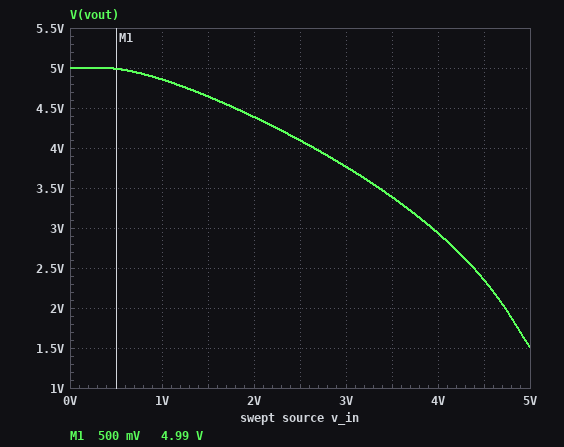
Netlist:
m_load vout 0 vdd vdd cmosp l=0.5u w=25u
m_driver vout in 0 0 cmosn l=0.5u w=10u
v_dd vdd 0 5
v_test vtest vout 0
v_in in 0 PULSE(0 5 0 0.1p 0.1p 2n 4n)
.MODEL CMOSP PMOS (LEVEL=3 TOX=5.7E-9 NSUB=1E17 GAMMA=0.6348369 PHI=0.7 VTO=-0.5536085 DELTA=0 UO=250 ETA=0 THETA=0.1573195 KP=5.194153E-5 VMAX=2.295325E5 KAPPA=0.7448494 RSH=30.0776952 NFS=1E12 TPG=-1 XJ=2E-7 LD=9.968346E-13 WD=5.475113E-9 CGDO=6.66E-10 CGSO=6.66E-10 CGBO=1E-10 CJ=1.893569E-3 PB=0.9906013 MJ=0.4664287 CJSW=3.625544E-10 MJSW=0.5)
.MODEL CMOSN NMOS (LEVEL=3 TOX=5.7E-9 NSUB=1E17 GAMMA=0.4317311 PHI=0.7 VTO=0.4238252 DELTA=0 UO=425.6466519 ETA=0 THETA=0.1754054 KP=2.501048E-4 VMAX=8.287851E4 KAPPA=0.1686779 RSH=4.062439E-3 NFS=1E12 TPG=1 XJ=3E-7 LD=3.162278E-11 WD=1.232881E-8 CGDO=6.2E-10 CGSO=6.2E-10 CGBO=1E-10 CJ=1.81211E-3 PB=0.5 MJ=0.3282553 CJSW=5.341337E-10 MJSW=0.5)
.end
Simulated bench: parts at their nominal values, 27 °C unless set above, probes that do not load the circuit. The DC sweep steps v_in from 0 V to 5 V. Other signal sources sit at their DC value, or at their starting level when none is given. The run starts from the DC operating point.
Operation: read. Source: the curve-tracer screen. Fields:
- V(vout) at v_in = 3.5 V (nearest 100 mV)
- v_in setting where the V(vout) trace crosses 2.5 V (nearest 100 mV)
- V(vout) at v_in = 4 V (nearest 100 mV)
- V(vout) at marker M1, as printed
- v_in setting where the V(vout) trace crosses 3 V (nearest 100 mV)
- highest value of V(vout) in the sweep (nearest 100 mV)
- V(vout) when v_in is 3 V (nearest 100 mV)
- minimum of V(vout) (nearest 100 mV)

3.4 V
4.4 V
2.9 V
4.99 V
3.9 V
5.0 V
3.8 V
1.5 V
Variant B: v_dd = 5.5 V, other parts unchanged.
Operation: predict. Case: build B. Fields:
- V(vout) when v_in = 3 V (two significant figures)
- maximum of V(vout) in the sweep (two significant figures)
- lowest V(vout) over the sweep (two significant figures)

4.3 V
5.5 V
2.6 V
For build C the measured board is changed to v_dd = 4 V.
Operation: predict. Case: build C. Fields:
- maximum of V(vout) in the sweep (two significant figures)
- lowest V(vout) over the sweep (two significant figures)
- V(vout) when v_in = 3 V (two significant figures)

4.0 V
730 mV
2.5 V
